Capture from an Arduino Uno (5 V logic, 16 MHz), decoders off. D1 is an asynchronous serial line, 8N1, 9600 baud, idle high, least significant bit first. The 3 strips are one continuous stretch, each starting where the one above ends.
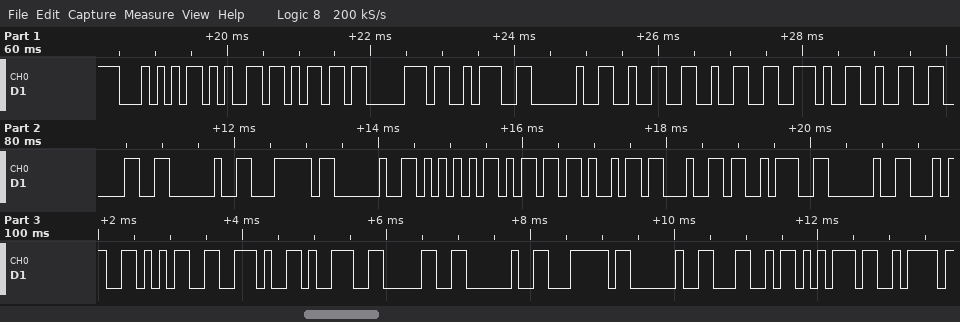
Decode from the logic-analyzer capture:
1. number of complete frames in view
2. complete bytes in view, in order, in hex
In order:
31
0x54 0x65 0x6D 0x70 0x3A 0x20 0x32 0x32 0x2E 0x32 0x30 0x20 0x7C 0x20 0x55 0x6D 0x69 0x64 0x3A 0x20 0x34 0x35 0x2E 0x39 0x30 0x20 0x7C 0x20 0x4C 0x75 0x7A
